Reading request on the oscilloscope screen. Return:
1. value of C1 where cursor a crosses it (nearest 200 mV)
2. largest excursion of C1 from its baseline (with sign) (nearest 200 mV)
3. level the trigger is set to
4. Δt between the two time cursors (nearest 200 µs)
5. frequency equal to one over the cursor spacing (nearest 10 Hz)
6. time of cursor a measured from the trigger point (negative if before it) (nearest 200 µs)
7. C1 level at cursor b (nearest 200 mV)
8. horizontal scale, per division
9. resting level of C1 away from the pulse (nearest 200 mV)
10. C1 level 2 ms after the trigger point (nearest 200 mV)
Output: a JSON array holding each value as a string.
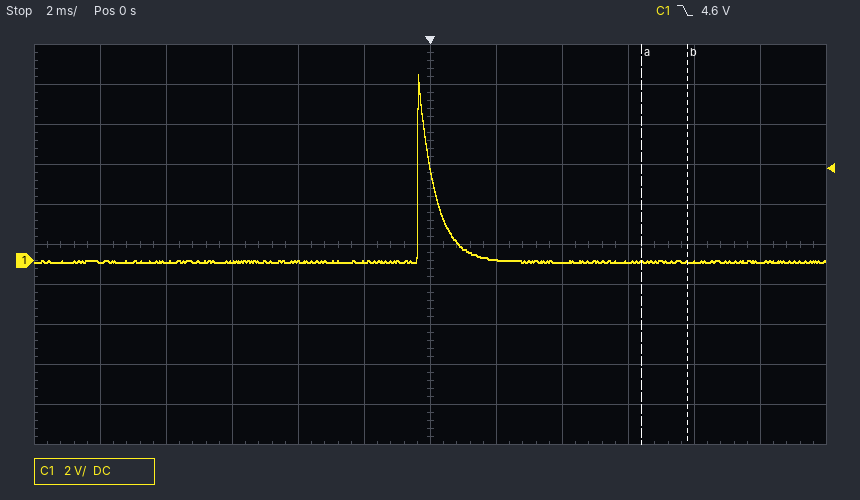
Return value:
["0.0 V", "+9.4 V", "4.6 V", "1.4 ms", "710 Hz", "+6.4 ms", "0.0 V", "2 ms", "0.0 V", "0.0 V"]
